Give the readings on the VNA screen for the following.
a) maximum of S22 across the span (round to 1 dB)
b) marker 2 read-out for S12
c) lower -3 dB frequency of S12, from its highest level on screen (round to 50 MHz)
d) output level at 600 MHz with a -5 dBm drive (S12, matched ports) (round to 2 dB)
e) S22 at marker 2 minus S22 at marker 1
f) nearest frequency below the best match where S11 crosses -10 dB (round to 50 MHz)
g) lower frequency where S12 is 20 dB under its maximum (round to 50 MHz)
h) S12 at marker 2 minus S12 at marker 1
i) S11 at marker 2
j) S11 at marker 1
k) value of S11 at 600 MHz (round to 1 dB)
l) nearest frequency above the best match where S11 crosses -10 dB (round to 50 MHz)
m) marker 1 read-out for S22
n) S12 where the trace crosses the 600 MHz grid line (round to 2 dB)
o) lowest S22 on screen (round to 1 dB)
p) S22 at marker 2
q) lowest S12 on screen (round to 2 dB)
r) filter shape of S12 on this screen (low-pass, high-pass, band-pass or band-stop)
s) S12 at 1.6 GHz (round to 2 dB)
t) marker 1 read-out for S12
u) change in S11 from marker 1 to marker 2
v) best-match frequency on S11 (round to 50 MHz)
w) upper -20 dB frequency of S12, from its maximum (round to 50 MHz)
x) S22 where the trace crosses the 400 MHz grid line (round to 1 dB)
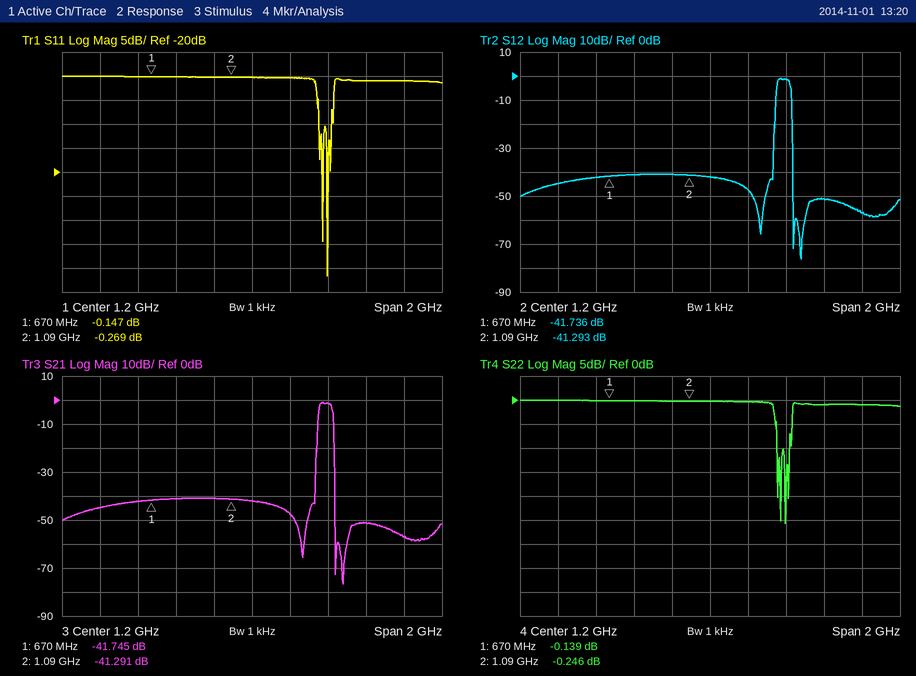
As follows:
0 dB
-41.293 dB
1.55 GHz
-48 dBm
-0.107 dB
1.55 GHz
1.55 GHz
0.443 dB
-0.269 dB
-0.147 dB
0 dB
1.60 GHz
-0.139 dB
-42 dB
-26 dB
-0.246 dB
-76 dB
band-pass
-2 dB
-41.736 dB
-0.122 dB
1.60 GHz
1.65 GHz
0 dB
